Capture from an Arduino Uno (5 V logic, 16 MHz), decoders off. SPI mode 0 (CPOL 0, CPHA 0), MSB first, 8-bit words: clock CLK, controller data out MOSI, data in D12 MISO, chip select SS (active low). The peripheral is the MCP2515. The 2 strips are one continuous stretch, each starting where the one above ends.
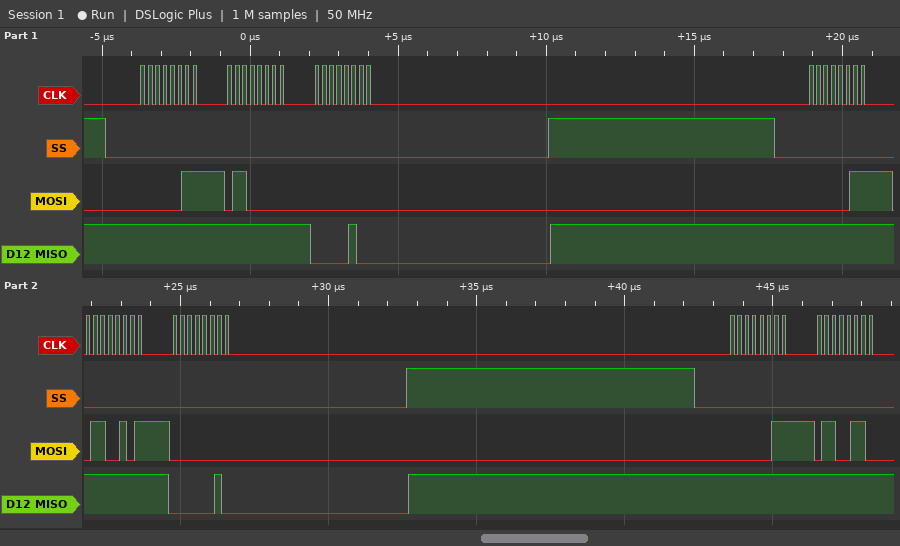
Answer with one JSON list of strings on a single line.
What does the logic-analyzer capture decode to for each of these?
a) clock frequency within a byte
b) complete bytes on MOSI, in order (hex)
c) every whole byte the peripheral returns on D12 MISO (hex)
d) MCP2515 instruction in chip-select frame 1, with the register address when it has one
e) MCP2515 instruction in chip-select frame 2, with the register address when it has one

["4 MHz", "03 60 00 03 65 00 03 66", "FF FF 04 FF FF 02 FF FF", "READ 0x60", "READ 0x65"]
